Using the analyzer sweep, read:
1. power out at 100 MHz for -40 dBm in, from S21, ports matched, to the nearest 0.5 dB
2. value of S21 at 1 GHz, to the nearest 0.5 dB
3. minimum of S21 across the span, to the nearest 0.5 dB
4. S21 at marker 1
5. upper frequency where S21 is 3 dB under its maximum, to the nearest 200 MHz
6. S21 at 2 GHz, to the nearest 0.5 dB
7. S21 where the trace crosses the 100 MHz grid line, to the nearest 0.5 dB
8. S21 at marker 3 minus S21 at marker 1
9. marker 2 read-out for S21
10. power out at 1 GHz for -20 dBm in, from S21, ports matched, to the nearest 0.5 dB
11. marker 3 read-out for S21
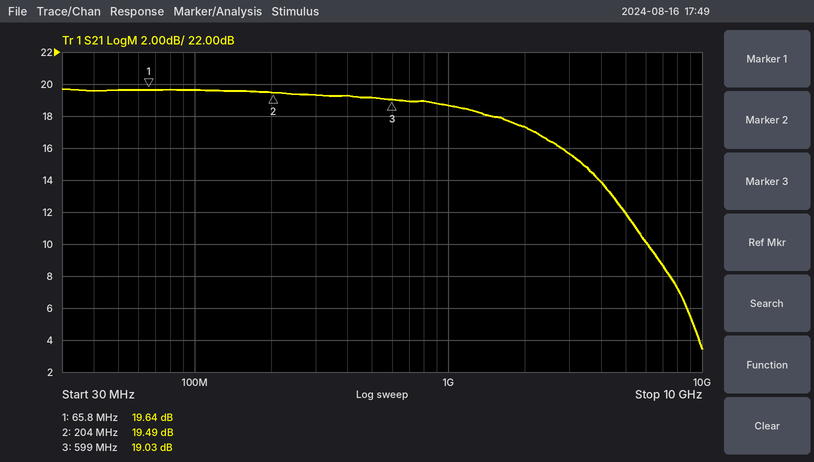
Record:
-20.5 dBm
18.5 dB
3.5 dB
19.64 dB
2.4 GHz
17.5 dB
19.5 dB
-0.61 dB
19.49 dB
-1.5 dBm
19.03 dB
